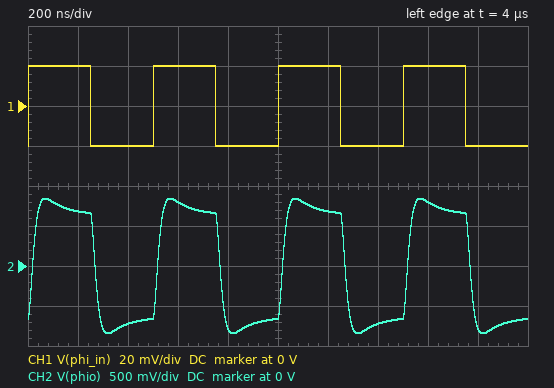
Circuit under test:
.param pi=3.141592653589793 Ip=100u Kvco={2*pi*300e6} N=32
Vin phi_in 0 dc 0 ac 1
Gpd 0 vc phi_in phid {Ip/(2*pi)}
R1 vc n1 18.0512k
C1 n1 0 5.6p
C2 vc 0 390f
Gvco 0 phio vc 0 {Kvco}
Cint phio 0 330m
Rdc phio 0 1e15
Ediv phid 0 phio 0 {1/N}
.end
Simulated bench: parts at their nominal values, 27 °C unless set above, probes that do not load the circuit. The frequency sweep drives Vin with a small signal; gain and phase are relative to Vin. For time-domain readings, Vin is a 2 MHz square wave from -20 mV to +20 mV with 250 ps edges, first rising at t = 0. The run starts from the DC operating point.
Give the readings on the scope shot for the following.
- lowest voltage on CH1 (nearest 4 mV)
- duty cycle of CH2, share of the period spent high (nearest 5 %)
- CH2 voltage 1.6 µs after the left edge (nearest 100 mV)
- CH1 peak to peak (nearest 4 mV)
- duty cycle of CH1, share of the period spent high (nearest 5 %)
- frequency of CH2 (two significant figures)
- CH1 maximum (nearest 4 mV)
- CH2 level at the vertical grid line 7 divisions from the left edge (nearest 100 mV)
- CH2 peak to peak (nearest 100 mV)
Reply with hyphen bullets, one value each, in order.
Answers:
- -20 mV
- 50 %
- 800 mV
- 40 mV
- 50 %
- 2.0 MHz
- 20 mV
- -700 mV
- 1.7 V
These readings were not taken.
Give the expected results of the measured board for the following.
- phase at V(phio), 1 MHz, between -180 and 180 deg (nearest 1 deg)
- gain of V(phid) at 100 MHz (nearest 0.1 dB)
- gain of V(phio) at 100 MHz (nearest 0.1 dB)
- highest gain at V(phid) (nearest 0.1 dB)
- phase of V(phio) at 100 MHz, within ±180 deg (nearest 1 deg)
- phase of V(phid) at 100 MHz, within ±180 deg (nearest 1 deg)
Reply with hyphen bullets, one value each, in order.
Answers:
- -2 deg
- -34.8 dB
- -4.7 dB
- 1.4 dB
- -167 deg
- -167 deg
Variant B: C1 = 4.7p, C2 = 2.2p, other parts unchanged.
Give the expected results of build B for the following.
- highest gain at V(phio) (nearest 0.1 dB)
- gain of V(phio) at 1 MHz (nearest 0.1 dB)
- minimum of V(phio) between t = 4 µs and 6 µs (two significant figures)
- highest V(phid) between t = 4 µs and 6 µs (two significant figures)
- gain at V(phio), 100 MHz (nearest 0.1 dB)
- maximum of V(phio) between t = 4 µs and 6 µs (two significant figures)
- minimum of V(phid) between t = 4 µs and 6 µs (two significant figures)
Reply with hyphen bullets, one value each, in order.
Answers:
- 36.1 dB
- 30.8 dB
- -1.3 V
- 40 mV
- -19.6 dB
- 1.3 V
- -40 mV
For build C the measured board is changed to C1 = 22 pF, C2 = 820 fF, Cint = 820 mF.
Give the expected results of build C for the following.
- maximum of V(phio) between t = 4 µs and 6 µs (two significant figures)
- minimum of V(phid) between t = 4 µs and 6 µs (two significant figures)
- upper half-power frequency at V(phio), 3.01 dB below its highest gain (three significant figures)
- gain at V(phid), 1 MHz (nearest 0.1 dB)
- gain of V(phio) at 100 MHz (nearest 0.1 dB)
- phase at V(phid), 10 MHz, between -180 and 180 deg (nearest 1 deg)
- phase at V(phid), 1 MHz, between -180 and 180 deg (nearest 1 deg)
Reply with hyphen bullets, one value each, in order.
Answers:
- 730 mV
- -23 mV
- 4.00 MHz
- 0.9 dB
- -19.0 dB
- -123 deg
- -17 deg
